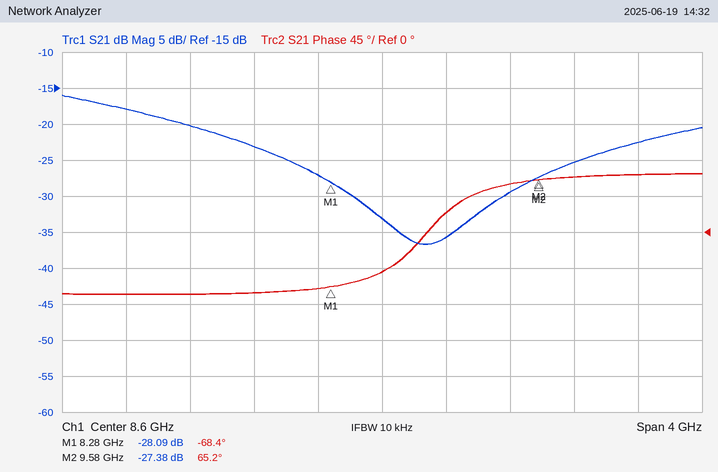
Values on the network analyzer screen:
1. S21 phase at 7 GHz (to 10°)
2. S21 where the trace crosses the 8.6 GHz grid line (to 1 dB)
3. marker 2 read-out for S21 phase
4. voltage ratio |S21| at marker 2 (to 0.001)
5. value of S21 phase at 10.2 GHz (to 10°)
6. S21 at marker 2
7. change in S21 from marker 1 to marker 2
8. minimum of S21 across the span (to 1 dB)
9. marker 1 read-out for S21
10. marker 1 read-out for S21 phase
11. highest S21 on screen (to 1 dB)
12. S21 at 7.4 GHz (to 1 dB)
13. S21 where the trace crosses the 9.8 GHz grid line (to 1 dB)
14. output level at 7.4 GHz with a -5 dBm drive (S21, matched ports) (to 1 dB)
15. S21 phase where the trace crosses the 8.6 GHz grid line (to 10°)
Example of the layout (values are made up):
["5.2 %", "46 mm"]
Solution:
["-80°", "-33 dB", "65.2°", "0.043", "70°", "-27.38 dB", "0.71 dB", "-37 dB", "-28.09 dB", "-68.4°", "-16 dB", "-20 dB", "-25 dB", "-25 dBm", "-50°"]
